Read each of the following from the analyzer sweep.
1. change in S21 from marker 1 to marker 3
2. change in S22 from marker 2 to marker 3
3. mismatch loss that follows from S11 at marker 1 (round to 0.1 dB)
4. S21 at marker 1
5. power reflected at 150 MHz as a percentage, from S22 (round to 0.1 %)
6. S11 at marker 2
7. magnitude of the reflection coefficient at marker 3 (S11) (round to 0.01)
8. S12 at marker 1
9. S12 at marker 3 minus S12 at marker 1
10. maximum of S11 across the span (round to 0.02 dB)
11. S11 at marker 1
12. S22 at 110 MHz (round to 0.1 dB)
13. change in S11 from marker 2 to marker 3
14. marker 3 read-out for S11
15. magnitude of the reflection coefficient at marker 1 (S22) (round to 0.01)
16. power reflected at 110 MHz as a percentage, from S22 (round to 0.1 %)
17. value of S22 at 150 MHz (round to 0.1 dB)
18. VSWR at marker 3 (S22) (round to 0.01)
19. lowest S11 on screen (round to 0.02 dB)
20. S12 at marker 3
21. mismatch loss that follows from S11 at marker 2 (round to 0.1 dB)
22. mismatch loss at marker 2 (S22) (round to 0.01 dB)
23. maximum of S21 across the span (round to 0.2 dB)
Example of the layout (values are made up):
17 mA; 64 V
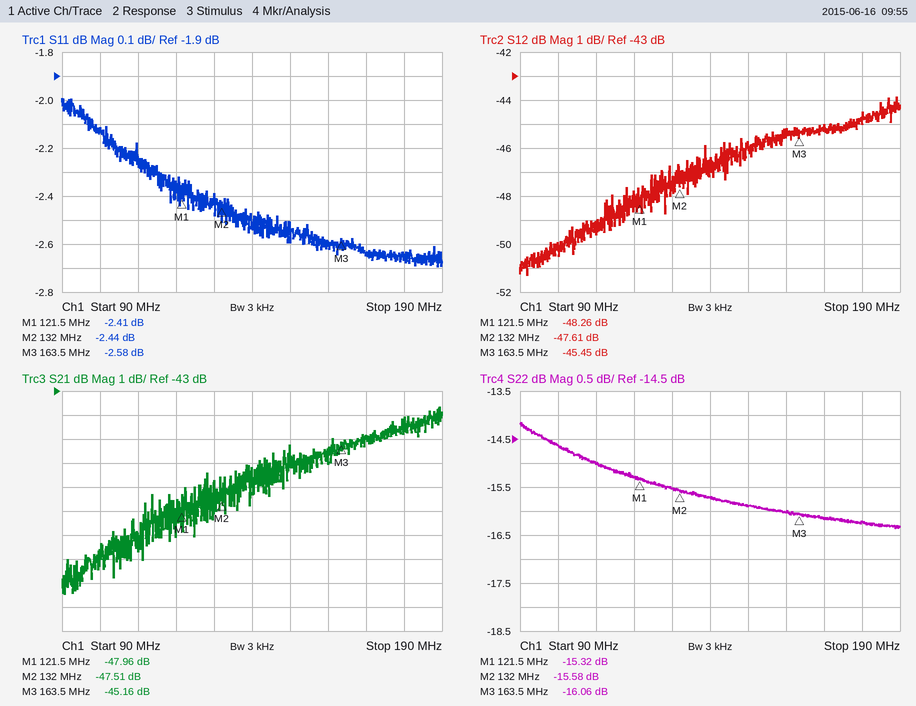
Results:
2.80 dB; -0.48 dB; 3.7 dB; -47.96 dB; 2.6 %; -2.44 dB; 0.74; -48.26 dB; 2.81 dB; -2.00 dB; -2.41 dB; -15.0 dB; -0.14 dB; -2.58 dB; 0.17; 3.2 %; -15.9 dB; 1.37; -2.70 dB; -45.45 dB; 3.7 dB; 0.12 dB; -43.6 dB
